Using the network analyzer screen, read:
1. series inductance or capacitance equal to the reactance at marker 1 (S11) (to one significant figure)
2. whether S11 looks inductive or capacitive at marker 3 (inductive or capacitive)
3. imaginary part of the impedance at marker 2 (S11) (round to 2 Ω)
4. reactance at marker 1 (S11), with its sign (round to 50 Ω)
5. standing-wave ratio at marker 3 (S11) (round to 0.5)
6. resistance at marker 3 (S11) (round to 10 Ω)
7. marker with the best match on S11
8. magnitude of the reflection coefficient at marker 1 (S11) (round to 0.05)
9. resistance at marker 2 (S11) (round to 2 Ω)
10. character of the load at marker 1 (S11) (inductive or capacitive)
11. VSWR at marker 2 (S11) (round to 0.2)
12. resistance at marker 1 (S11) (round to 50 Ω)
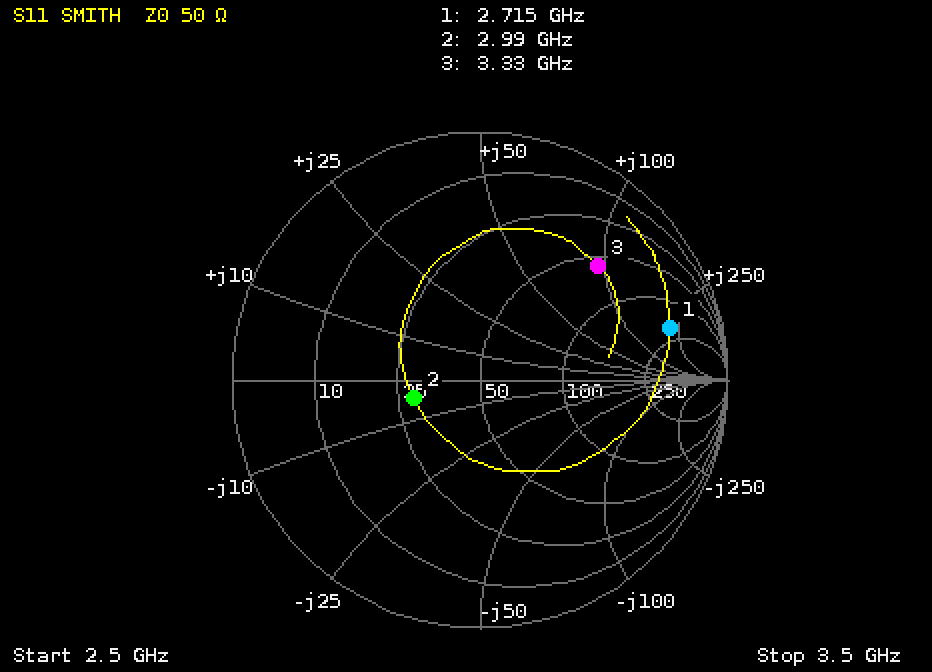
10 nH
inductive
-4 Ω
+200 Ω
5.0
60 Ω
marker 2
0.80
28 Ω
inductive
1.8
200 Ω
